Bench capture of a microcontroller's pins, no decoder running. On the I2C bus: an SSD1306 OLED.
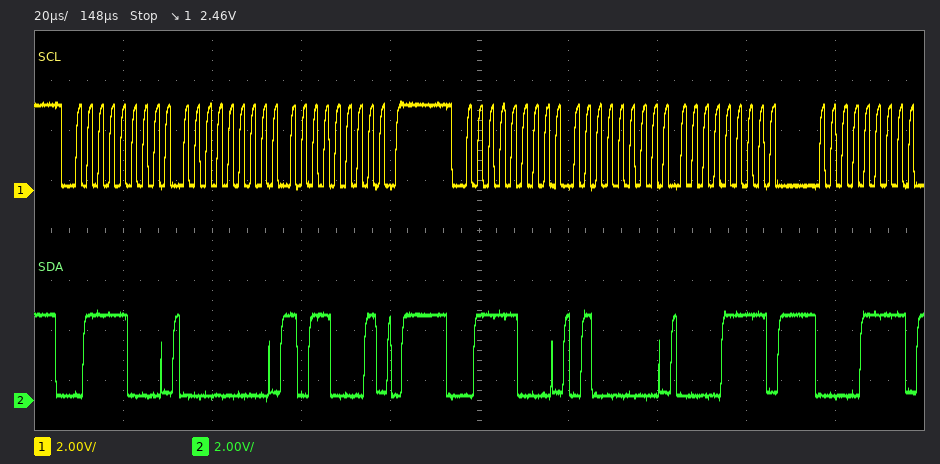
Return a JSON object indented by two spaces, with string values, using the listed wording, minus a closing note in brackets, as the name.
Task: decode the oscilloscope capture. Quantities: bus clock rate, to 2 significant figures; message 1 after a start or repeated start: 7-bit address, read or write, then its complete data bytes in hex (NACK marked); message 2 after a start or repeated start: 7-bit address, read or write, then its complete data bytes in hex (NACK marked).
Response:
{
  "bus clock rate, to 2 significant figures": "400 kHz",
  "message 1 after a start or repeated start: 7-bit address, read or write, then its complete data bytes in hex": "0x3C write: 00 B1",
  "message 2 after a start or repeated start: 7-bit address, read or write, then its complete data bytes in hex": "0x3C write: 40 0F 0F"
}
